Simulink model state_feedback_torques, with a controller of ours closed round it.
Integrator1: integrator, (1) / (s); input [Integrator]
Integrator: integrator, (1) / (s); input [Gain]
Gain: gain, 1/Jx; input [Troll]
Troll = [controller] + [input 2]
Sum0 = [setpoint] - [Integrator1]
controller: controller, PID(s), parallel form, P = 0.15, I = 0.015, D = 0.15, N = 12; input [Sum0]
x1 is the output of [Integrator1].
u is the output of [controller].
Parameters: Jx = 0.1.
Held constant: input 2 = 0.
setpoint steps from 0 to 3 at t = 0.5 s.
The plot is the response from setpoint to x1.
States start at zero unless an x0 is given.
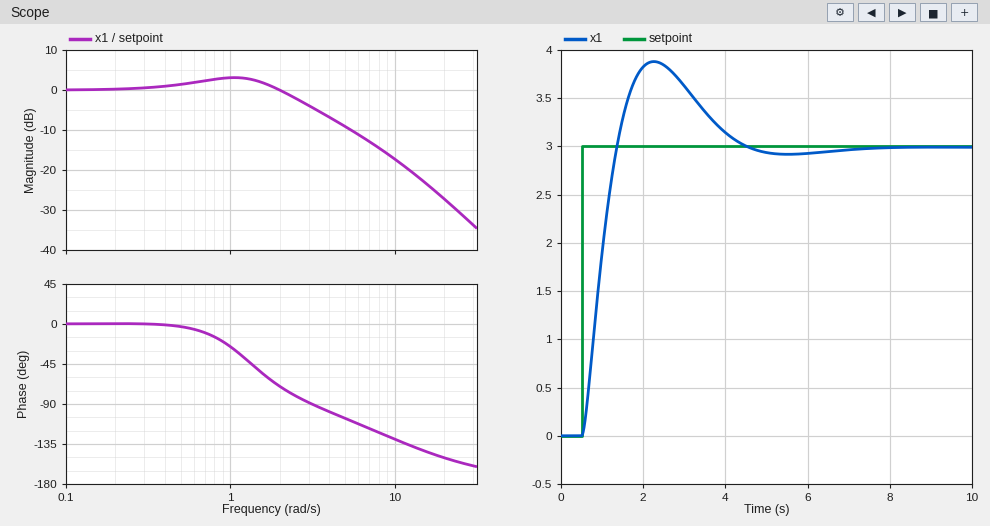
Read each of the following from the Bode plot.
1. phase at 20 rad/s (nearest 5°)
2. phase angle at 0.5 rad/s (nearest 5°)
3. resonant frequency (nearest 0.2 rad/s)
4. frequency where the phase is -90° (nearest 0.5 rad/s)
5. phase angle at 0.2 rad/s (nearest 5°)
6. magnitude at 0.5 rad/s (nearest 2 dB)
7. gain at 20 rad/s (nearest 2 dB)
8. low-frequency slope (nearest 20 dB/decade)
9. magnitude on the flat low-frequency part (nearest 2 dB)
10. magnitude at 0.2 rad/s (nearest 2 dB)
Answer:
-150°
-5°
1.0 rad/s
3.0 rad/s
0°
2 dB
-28 dB
0 dB/decade
0 dB
0 dB
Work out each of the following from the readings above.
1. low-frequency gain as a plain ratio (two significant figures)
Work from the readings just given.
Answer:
1.0
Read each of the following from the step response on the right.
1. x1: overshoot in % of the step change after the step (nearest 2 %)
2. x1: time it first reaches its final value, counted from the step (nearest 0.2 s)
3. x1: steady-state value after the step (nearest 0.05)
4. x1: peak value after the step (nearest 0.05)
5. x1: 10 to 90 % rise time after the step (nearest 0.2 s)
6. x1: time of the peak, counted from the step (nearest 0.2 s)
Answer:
30 %
0.8 s
3.00
3.90
0.6 s
1.8 s
